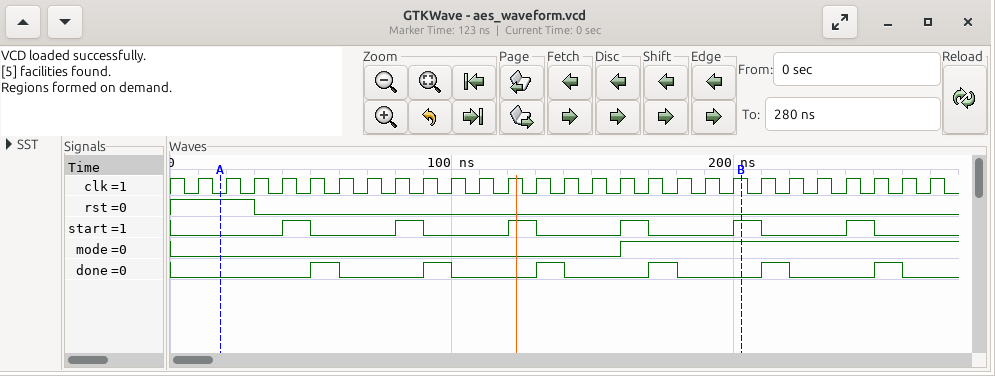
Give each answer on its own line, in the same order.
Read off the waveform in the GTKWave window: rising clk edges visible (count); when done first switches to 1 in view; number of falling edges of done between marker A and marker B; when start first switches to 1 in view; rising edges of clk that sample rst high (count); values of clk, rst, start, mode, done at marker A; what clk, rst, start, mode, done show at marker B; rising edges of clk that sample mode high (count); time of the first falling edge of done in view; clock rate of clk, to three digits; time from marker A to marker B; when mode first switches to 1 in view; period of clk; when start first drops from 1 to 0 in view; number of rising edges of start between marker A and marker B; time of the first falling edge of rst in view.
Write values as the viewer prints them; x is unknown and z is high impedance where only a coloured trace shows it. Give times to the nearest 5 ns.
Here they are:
27
50 ns
4
40 ns
3
clk=0, rst=1, start=0, mode=0, done=0
clk=1, rst=0, start=1, mode=1, done=0
11
60 ns
100 MHz
185 ns
160 ns
10 ns
50 ns
5
30 ns
